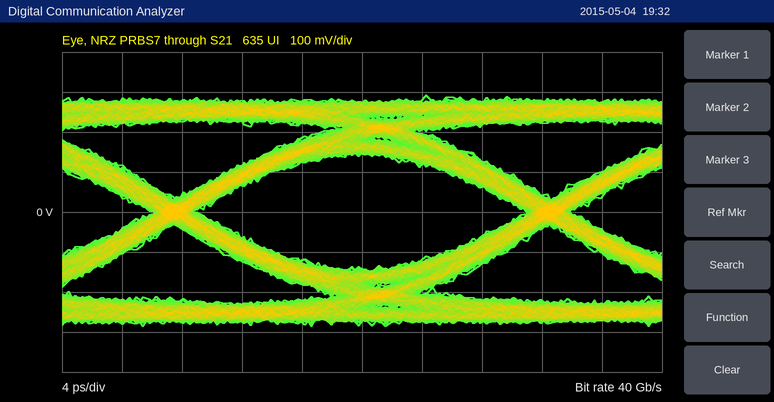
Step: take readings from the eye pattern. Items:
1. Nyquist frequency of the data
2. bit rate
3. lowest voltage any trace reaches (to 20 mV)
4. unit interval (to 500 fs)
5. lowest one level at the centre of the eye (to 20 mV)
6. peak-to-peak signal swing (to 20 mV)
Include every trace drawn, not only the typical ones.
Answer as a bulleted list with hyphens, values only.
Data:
- 20 GHz
- 40 Gb/s
- -280 mV
- 25.0 ps
- 140 mV
- 580 mV
